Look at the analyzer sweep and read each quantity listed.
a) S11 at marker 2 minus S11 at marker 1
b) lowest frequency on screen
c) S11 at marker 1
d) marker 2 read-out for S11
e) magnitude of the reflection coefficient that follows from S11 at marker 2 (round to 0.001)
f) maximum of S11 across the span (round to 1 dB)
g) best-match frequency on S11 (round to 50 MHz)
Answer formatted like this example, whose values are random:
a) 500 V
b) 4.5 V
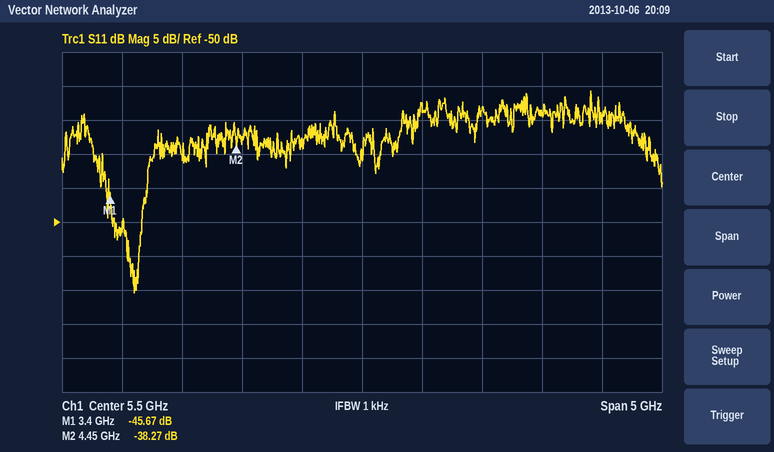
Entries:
a) 7.40 dB
b) 3 GHz
c) -45.67 dB
d) -38.27 dB
e) 0.012
f) -31 dB
g) 3.60 GHz
